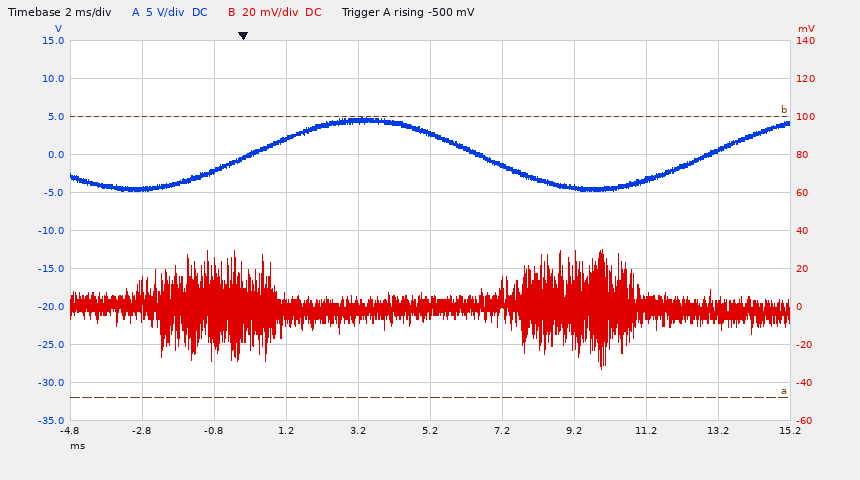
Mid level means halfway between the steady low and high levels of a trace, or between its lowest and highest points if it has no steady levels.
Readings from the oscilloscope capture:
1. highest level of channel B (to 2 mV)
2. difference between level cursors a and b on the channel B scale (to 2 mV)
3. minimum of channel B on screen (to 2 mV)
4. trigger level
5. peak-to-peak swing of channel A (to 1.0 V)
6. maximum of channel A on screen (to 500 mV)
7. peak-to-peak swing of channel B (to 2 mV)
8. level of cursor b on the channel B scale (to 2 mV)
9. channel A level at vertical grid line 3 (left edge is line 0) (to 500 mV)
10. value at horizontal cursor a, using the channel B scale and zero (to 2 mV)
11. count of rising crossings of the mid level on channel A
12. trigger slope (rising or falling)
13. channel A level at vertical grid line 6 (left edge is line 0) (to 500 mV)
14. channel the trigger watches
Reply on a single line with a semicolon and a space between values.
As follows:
30 mV; 148 mV; -32 mV; -500 mV; 10.0 V; 5.0 V; 62 mV; 100 mV; 2.0 V; -48 mV; 2; rising; -1.5 V; channel A
